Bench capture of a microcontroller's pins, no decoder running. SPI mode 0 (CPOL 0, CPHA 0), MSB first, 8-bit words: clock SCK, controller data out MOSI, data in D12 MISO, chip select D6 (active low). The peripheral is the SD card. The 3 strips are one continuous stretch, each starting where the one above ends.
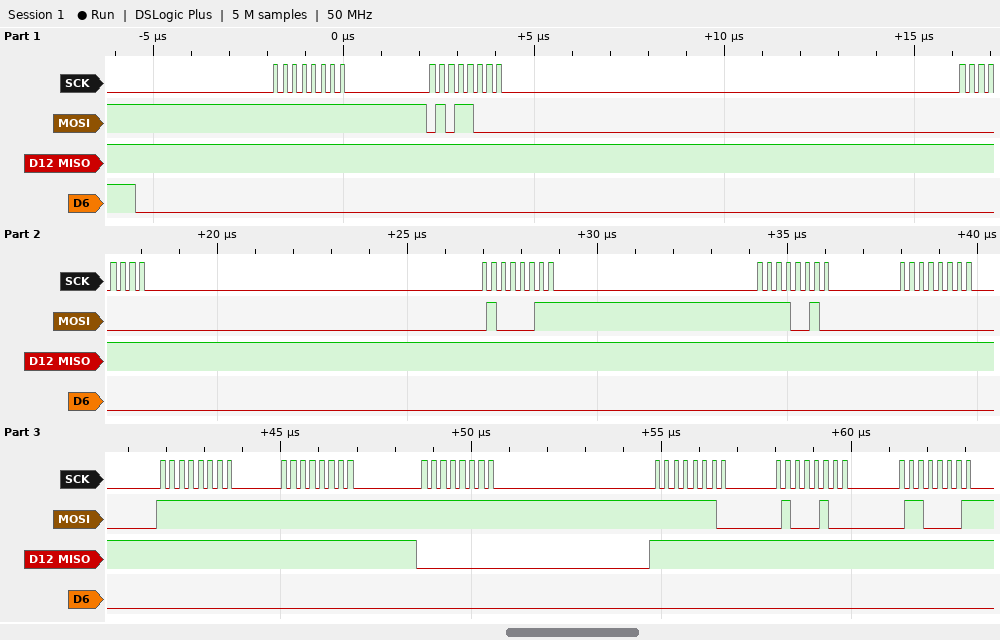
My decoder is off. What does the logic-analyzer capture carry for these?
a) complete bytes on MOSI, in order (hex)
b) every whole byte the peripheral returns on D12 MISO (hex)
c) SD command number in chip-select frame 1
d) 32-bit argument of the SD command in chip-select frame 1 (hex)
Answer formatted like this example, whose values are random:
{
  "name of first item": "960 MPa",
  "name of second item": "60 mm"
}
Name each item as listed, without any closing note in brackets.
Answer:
{
  "complete bytes on MOSI, in order": "0xFF 0x58 0x00 0x43 0xF2 0x00 0xFF 0xFF 0xFF 0xFE 0x44 0x61",
  "every whole byte the peripheral returns on D12 MISO": "0xFF 0xFF 0xFF 0xFF 0xFF 0xFF 0xFF 0xFF 0x00 0xFF 0xFF 0xFF",
  "SD command number in chip-select frame 1": "CMD24",
  "32-bit argument of the SD command in chip-select frame 1": "0x0043F200"
}
